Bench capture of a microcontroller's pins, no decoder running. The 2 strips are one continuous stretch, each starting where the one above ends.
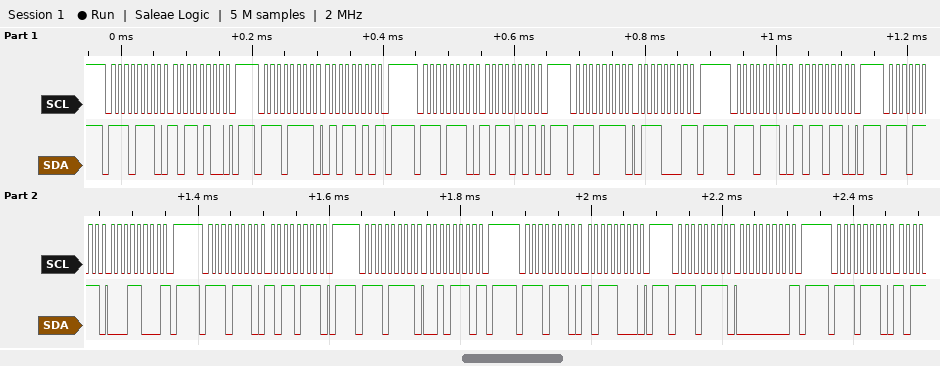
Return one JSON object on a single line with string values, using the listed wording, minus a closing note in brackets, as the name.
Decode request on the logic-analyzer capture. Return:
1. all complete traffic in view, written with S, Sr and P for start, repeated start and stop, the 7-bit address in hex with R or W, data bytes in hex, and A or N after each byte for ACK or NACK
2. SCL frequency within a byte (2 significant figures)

{"all complete traffic in view, written with S, Sr and P for start, repeated start and stop, the 7-bit address in hex with R or W, data bytes in hex, and A or N after each byte for ACK or NACK": "S 77W A B4 A P S 77R A 5A N P S 77W A B5 A P S 77R A 71 N P S 77W A B6 A P S 77R A 18 N P S 77W A B7 A P S 77R A 2E N P S 77W A B8 A P S 77R A 00 N P S 77W A", "SCL frequency within a byte": "100 kHz"}
